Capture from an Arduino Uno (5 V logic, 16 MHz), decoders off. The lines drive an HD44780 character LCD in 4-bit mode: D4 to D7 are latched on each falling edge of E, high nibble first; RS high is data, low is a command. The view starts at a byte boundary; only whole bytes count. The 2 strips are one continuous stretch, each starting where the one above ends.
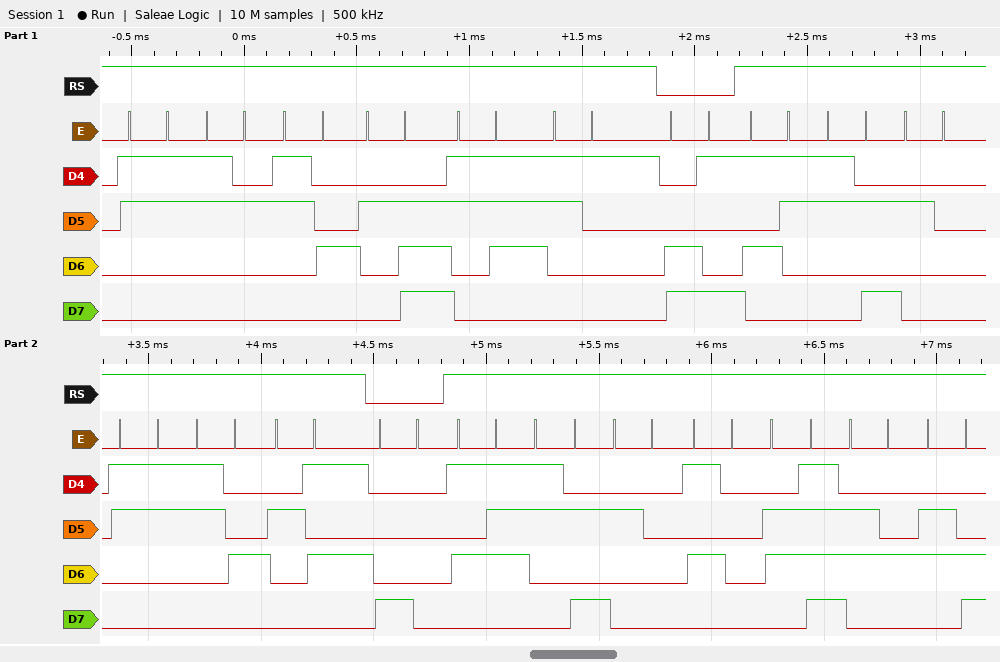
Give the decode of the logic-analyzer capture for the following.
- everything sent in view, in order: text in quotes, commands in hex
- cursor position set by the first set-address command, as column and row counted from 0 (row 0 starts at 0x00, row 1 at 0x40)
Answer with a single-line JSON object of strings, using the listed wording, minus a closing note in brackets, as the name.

{"everything sent in view, in order: text in quotes, commands in hex": "\"324.71\" 0xC9 \"S: 34%\" 0x80 \"W: Podl\"", "cursor position set by the first set-address command, as column and row counted from 0": "column 9, row 1"}
